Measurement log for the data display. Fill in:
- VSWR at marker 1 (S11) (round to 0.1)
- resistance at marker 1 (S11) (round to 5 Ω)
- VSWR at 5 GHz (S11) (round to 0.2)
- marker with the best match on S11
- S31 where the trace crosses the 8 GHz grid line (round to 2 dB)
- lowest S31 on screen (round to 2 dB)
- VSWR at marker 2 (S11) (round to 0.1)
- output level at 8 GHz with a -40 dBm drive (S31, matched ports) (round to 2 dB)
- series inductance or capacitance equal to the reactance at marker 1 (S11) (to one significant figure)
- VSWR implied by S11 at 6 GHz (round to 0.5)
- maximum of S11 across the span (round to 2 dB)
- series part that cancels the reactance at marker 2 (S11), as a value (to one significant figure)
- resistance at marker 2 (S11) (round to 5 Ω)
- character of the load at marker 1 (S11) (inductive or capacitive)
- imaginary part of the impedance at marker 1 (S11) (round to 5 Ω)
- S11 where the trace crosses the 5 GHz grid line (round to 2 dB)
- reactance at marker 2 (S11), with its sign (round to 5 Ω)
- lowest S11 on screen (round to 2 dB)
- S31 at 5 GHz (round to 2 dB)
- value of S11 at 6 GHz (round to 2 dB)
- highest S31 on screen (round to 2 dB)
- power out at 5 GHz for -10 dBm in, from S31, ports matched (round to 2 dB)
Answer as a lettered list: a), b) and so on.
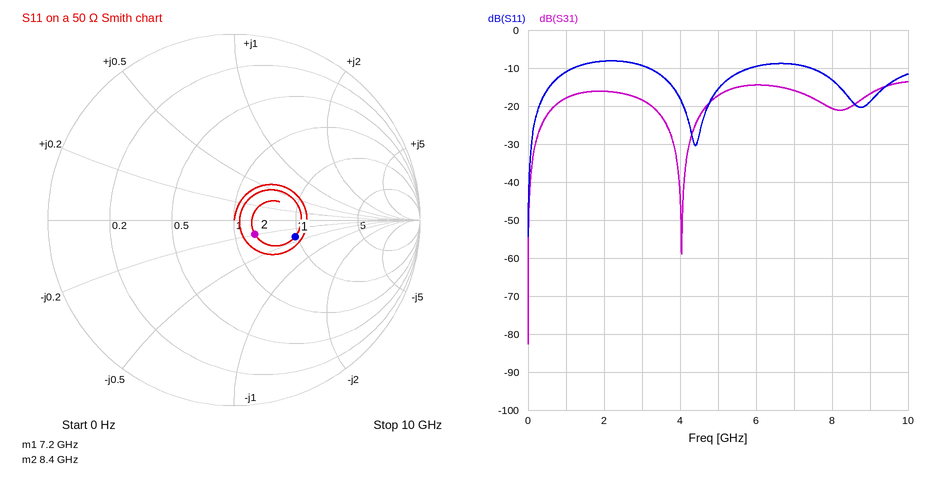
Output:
a) 2.0
b) 95 Ω
c) 1.4
d) marker 2
e) -20 dB
f) -82 dB
g) 1.3
h) -60 dBm
i) 1 pF
j) 2.0
k) -8 dB
l) 200 pH
m) 60 Ω
n) capacitive
o) -20 Ω
p) -16 dB
q) -10 Ω
r) -54 dB
s) -18 dB
t) -10 dB
u) -14 dB
v) -28 dBm
